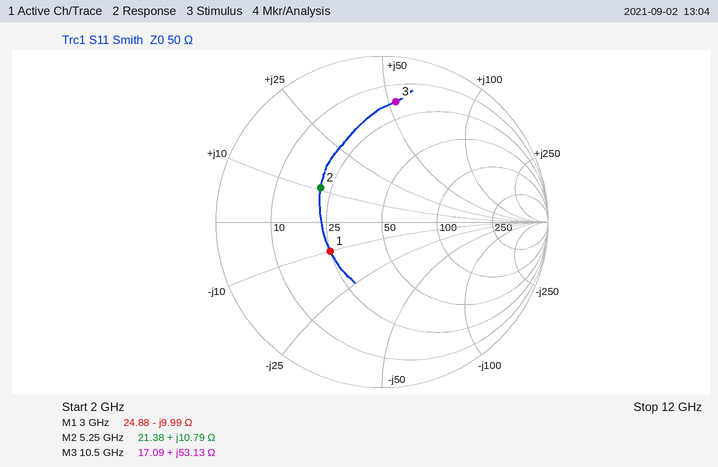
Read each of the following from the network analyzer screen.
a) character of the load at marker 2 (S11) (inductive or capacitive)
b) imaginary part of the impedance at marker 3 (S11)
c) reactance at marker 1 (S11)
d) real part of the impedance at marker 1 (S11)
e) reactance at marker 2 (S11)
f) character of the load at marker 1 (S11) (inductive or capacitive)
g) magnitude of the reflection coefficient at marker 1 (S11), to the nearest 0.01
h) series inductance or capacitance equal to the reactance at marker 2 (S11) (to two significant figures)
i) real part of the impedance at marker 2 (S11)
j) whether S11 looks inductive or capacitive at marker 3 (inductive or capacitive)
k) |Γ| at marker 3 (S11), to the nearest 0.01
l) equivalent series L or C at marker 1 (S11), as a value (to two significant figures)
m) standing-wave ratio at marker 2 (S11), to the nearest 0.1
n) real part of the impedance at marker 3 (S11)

inductive
+53.13 Ω
-9.99 Ω
24.88 Ω
+10.79 Ω
capacitive
0.36
330 pH
21.38 Ω
inductive
0.73
5.3 pF
2.5
17.09 Ω
